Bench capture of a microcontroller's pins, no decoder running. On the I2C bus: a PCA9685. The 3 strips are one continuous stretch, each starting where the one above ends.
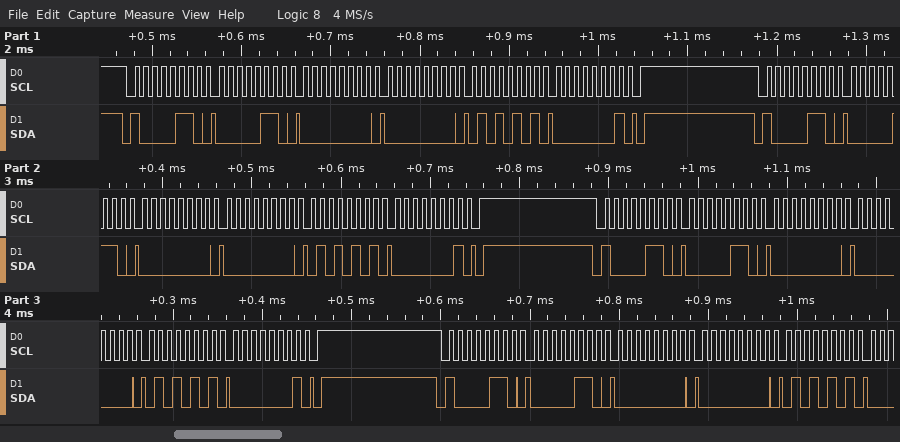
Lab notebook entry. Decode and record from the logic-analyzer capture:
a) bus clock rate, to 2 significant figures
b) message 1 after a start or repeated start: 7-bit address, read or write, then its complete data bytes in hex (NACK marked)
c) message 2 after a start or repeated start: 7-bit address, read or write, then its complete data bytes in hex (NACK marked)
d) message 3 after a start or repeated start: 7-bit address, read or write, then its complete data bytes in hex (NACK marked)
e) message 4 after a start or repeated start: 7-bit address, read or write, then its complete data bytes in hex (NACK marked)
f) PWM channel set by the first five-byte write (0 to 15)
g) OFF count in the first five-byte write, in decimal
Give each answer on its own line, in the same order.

100 kHz
0x43 write: 06 00 00 55 01
0x43 write: 06 00 00 55 01
0x43 write: 06 00 00 55 01
0x43 write: 06 00 00 55
0
341
